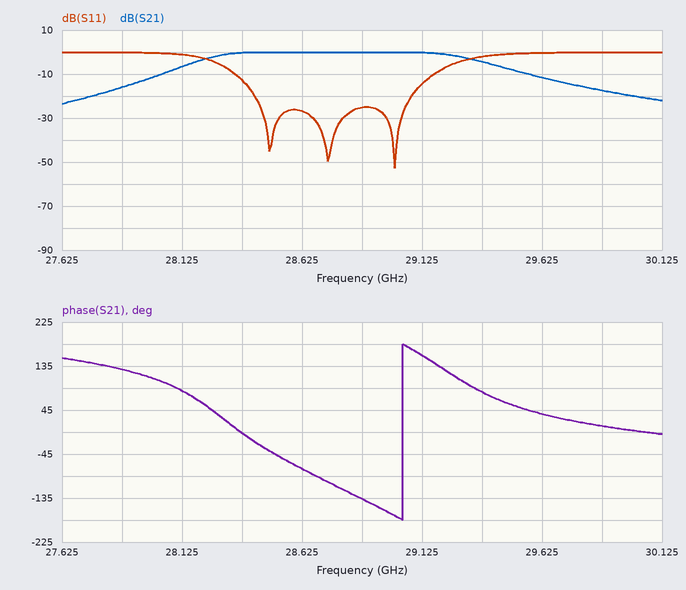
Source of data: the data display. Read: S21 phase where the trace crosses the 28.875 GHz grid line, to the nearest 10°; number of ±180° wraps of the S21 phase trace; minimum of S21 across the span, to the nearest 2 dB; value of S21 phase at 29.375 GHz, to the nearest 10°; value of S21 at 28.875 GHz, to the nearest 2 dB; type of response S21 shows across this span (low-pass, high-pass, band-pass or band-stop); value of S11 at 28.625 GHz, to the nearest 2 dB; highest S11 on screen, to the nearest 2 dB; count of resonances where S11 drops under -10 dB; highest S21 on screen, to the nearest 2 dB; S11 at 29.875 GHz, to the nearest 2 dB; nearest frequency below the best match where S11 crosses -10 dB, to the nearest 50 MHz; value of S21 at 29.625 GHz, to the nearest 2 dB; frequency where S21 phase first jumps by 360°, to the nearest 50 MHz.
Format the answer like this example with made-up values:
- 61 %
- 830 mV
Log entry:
- -140°
- 1
- -24 dB
- 80°
- 0 dB
- band-pass
- -26 dB
- 0 dB
- 3
- 0 dB
- 0 dB
- 28.35 GHz
- -12 dB
- 29.05 GHz
